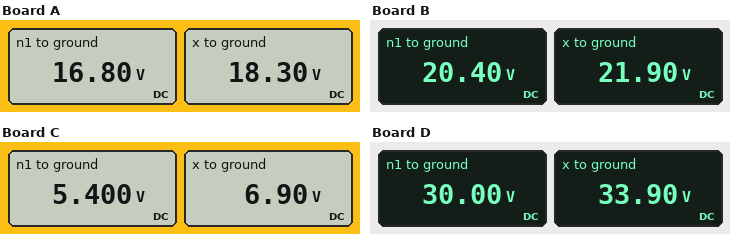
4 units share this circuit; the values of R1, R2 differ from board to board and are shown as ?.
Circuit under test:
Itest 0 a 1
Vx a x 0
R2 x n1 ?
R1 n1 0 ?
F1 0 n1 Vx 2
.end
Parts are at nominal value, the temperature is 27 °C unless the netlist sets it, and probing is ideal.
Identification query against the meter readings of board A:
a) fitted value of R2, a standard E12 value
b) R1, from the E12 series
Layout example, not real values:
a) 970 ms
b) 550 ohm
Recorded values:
a) 1.5 Ω
b) 5.6 Ω
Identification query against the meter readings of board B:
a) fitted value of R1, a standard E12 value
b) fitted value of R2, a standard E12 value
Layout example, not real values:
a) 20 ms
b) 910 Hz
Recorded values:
a) 6.8 Ω
b) 1.5 Ω
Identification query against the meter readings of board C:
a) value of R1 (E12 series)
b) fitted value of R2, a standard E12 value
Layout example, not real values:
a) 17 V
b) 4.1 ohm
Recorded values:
a) 1.8 Ω
b) 1.5 Ω
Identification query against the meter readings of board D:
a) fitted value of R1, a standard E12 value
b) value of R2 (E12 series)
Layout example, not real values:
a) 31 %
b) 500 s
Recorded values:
a) 10 Ω
b) 3.9 Ω
